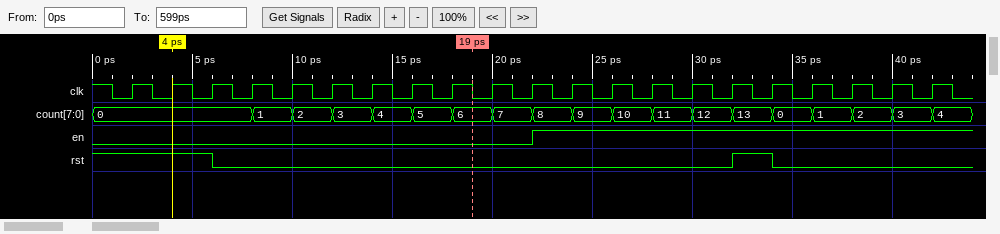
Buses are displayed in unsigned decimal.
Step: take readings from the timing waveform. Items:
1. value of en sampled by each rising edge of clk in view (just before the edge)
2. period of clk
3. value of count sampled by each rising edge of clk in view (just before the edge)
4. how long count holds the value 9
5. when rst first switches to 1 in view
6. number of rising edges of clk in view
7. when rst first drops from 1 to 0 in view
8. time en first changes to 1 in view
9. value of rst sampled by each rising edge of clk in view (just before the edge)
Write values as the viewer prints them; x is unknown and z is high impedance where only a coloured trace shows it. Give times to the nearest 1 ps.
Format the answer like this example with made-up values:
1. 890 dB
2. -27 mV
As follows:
1. 0 0 0 0 0 0 0 0 0 0 0 1 1 1 1 1 1 1 1 1 1
2. 2 ps
3. 0, 0, 0, 0, 1, 2, 3, 4, 5, 6, 7, 8, 9, 10, 11, 12, 13, 0, 1, 2, 3
4. 2 ps
5. 32 ps
6. 21
7. 6 ps
8. 22 ps
9. 1 1 1 0 0 0 0 0 0 0 0 0 0 0 0 0 1 0 0 0 0
